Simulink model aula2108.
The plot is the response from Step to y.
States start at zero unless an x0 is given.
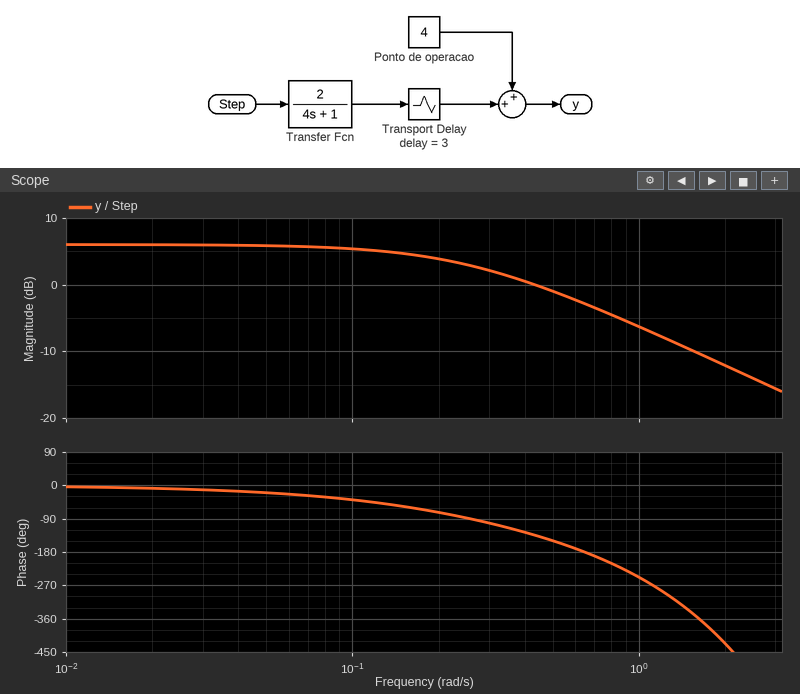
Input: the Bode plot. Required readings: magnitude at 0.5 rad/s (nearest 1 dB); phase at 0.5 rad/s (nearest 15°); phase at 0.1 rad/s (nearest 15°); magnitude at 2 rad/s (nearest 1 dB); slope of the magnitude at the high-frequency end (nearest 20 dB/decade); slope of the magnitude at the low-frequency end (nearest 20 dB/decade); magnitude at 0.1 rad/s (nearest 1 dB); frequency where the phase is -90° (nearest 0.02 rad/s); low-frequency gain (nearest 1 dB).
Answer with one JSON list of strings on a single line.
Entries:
["-1 dB", "-150°", "-45°", "-12 dB", "-20 dB/decade", "0 dB/decade", "5 dB", "0.26 rad/s", "6 dB"]
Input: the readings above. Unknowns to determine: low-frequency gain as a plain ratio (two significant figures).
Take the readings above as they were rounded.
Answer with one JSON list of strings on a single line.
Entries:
["2.0"]
